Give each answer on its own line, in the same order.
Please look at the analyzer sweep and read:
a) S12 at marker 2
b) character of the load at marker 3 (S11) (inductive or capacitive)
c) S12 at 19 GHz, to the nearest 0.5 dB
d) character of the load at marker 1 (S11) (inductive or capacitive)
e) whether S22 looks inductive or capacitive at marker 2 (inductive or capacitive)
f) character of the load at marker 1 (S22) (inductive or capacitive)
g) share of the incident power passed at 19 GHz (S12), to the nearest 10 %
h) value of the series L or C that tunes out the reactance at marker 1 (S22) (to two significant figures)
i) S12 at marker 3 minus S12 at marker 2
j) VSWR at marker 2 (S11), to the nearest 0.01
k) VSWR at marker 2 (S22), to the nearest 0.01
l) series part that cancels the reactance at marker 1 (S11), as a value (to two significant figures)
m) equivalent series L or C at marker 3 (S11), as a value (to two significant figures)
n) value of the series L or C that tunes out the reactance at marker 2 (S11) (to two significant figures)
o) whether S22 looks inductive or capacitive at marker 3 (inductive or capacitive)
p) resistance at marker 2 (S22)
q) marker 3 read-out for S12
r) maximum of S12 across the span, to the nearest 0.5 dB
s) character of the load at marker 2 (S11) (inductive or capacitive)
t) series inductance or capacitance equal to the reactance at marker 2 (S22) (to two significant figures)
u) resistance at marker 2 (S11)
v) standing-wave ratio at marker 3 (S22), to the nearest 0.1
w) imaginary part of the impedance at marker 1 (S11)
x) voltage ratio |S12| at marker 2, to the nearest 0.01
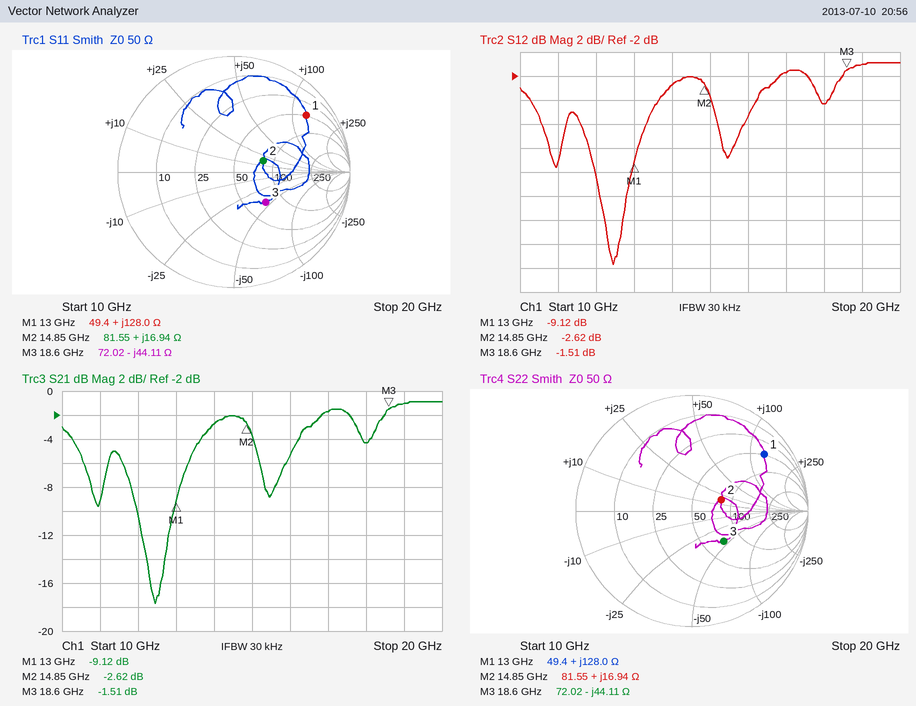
-2.62 dB
capacitive
-1.0 dB
inductive
inductive
inductive
80 %
96 fF
1.11 dB
1.74
1.74
96 fF
190 fF
630 fF
capacitive
81.55 Ω
-1.51 dB
-1.0 dB
inductive
180 pH
81.55 Ω
2.2
+128.0 Ω
0.74
